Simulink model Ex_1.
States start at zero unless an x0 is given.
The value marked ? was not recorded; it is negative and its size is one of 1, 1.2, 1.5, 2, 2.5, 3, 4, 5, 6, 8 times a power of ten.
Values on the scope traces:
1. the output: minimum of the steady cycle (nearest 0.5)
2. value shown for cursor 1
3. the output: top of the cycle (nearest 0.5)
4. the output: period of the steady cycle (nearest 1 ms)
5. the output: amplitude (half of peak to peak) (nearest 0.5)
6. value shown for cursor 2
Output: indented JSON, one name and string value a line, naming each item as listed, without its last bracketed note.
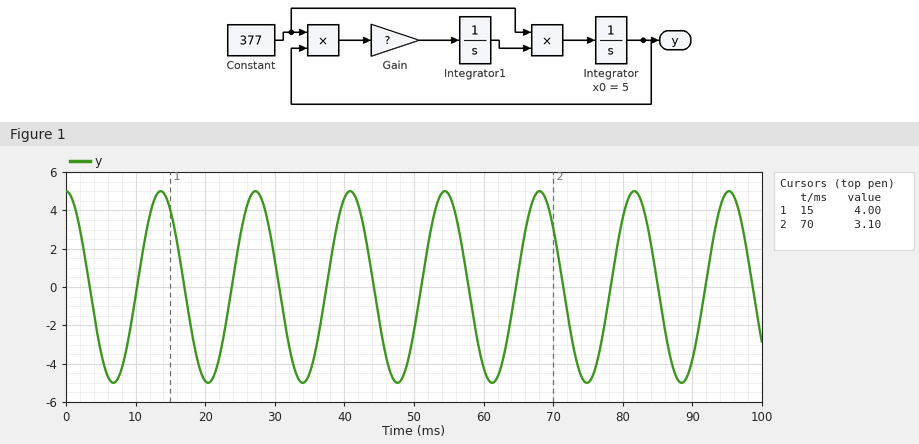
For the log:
{
  "the output: minimum of the steady cycle": "-5.0",
  "value shown for cursor 1": "4.00",
  "the output: top of the cycle": "5.0",
  "the output: period of the steady cycle": "14 ms",
  "the output: amplitude (half of peak to peak)": "5.0",
  "value shown for cursor 2": "3.10"
}
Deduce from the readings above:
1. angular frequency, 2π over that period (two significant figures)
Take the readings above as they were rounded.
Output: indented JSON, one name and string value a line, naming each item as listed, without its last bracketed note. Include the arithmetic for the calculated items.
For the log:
{
  "angular frequency, 2π over that period": "2π / 14 = 0.45 rad/ms"
}
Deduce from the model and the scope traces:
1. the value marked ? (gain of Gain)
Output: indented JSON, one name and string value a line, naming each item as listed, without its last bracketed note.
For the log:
{
  "the value marked ?": "-1.5"
}
